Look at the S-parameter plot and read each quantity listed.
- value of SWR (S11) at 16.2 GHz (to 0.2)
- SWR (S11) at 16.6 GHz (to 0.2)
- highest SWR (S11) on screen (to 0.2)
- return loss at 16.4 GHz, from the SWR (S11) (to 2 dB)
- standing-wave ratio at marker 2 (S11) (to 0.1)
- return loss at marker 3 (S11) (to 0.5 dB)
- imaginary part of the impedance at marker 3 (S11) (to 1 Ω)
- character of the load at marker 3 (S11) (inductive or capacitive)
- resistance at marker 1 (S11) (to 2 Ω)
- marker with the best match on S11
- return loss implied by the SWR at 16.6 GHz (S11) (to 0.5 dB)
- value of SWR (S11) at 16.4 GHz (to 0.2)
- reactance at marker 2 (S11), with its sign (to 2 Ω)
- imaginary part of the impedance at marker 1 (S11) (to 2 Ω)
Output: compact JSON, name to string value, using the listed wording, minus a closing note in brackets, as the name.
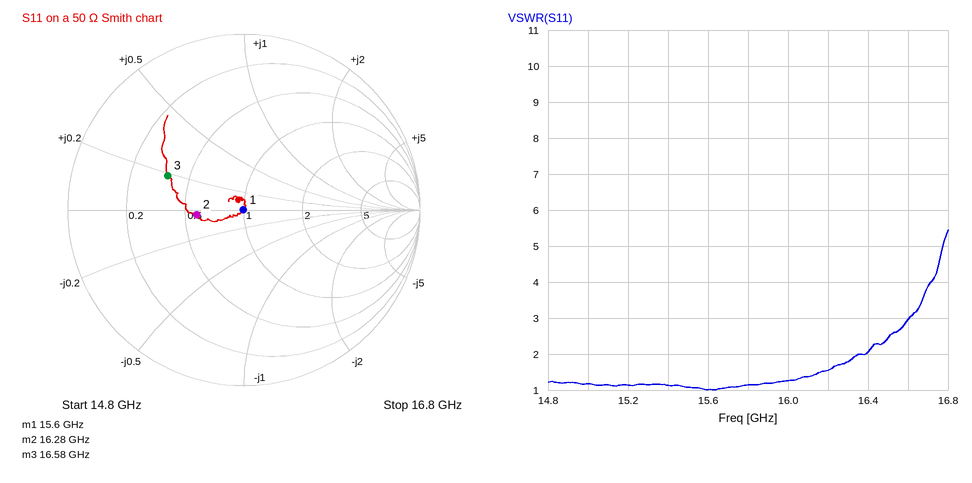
{"value of SWR (S11) at 16.2 GHz": "1.6", "SWR (S11) at 16.6 GHz": "3.0", "highest SWR (S11) on screen": "5.4", "return loss at 16.4 GHz, from the SWR (S11)": "10 dB", "standing-wave ratio at marker 2 (S11)": "1.7", "return loss at marker 3 (S11)": "6.5 dB", "imaginary part of the impedance at marker 3 (S11)": "+9 Ω", "character of the load at marker 3 (S11)": "inductive", "resistance at marker 1 (S11)": "50 Ω", "marker with the best match on S11": "marker 1", "return loss implied by the SWR at 16.6 GHz (S11)": "6.0 dB", "value of SWR (S11) at 16.4 GHz": "2.0", "reactance at marker 2 (S11), with its sign": "-2 Ω", "imaginary part of the impedance at marker 1 (S11)": "0 Ω"}
